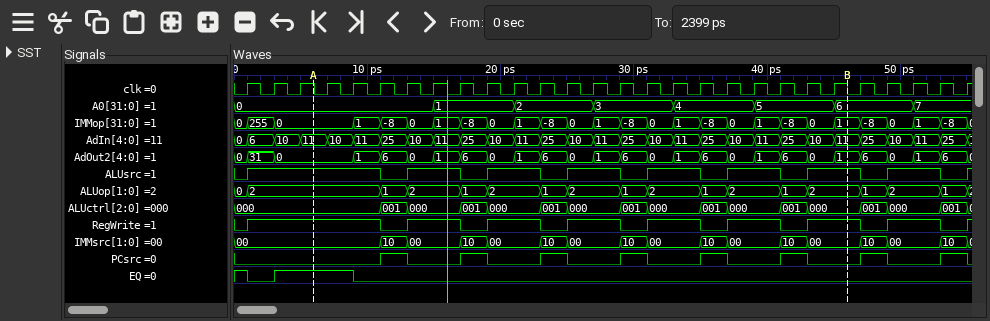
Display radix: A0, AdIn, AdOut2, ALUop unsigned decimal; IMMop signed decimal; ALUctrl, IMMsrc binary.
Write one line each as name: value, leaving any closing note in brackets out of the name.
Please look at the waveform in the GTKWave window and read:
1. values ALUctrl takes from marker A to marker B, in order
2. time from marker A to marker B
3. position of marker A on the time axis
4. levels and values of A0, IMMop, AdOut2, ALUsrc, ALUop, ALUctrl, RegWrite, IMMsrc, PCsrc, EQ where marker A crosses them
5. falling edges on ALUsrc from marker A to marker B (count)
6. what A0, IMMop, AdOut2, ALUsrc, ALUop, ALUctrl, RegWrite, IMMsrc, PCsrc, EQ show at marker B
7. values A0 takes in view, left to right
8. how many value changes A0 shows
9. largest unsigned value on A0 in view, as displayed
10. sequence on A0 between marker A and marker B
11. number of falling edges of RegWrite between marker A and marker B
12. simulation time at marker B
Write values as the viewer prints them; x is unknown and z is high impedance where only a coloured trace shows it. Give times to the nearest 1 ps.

values ALUctrl takes from marker A to marker B, in order: 000, 001, 000, 001, 000, 001, 000, 001, 000, 001, 000, 001, 000
time from marker A to marker B: 40 ps
position of marker A on the time axis: 6 ps
levels and values of A0, IMMop, AdOut2, ALUsrc, ALUop, ALUctrl, RegWrite, IMMsrc, PCsrc, EQ where marker A crosses them: A0=0, IMMop=0, AdOut2=0, ALUsrc=1, ALUop=2, ALUctrl=000, RegWrite=1, IMMsrc=00, PCsrc=0, EQ=1
falling edges on ALUsrc from marker A to marker B: 6
what A0, IMMop, AdOut2, ALUsrc, ALUop, ALUctrl, RegWrite, IMMsrc, PCsrc, EQ show at marker B: A0=6, IMMop=1, AdOut2=1, ALUsrc=1, ALUop=2, ALUctrl=000, RegWrite=1, IMMsrc=00, PCsrc=0, EQ=0
values A0 takes in view, left to right: 0, 1, 2, 3, 4, 5, 6, 7
how many value changes A0 shows: 7
largest unsigned value on A0 in view, as displayed: 7
sequence on A0 between marker A and marker B: 0, 1, 2, 3, 4, 5, 6
number of falling edges of RegWrite between marker A and marker B: 6
simulation time at marker B: 46 ps
